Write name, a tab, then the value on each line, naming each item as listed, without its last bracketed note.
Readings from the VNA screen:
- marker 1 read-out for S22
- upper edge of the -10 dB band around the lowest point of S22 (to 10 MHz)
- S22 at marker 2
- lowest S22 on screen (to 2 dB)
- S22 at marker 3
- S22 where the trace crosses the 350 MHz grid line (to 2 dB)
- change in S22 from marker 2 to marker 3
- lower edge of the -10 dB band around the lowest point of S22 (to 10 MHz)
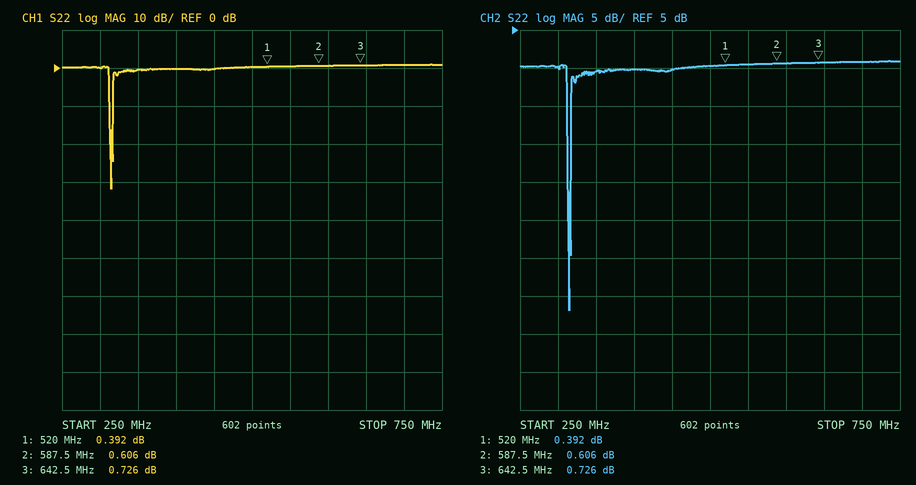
marker 1 read-out for S22	0.392 dB
upper edge of the -10 dB band around the lowest point of S22	320 MHz
S22 at marker 2	0.606 dB
lowest S22 on screen	-32 dB
S22 at marker 3	0.726 dB
S22 where the trace crosses the 350 MHz grid line	0 dB
change in S22 from marker 2 to marker 3	0.120 dB
lower edge of the -10 dB band around the lowest point of S22	310 MHz
